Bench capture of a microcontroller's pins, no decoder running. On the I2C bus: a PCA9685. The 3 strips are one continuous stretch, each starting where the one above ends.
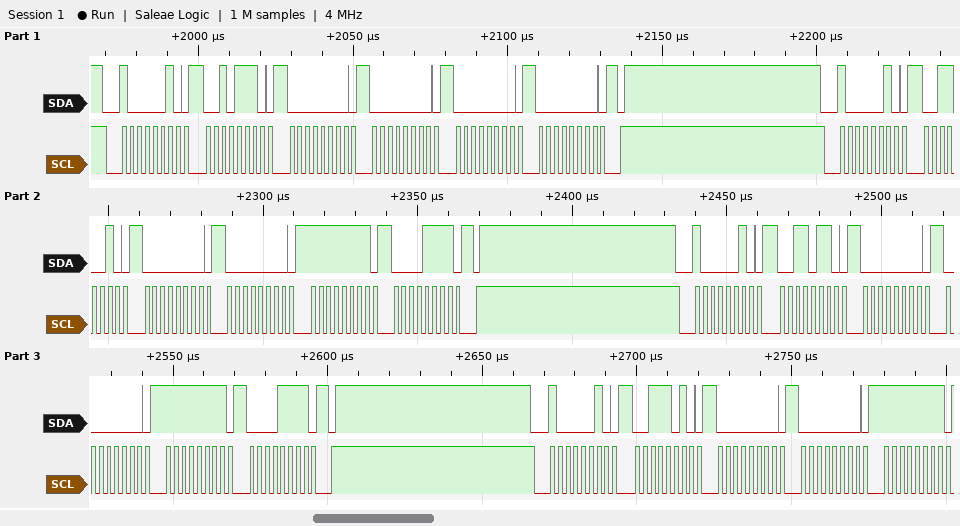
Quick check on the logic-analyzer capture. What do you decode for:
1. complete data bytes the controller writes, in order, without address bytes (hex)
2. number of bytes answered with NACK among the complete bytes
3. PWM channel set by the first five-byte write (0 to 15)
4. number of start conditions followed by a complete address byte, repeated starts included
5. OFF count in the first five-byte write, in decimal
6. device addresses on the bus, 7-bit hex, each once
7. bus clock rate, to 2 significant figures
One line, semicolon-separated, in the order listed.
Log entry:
2E 00 00 00 00 32 00 00 FF 0F 36 00 00 FF 0F 3A 00 00 FF; 0; 10; 4; 0; 0x41; 400 kHz
